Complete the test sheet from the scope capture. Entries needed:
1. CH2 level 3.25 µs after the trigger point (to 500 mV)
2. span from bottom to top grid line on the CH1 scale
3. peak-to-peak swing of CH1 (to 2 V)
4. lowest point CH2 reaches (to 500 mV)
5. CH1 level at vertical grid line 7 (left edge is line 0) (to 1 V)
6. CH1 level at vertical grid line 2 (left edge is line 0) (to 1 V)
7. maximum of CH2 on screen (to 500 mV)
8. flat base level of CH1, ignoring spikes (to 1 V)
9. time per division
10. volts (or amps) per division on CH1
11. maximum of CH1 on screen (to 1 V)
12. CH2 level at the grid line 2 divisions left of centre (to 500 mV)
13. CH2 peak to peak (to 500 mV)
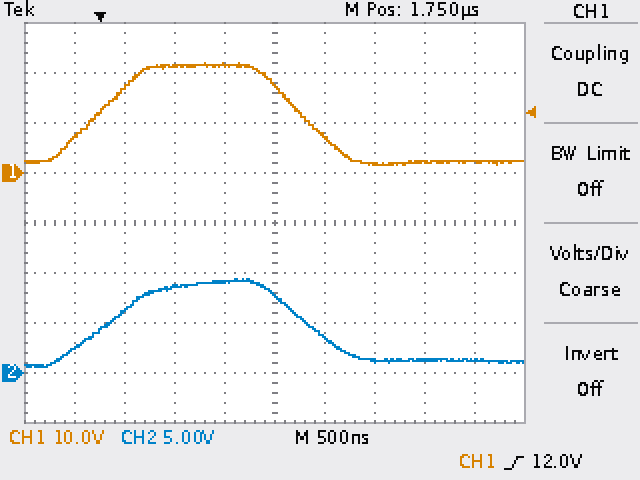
1.5 V
80 V
20 V
500 mV
2 V
17 V
9.5 V
2 V
500 ns
10 V
22 V
8.5 V
9.0 V
